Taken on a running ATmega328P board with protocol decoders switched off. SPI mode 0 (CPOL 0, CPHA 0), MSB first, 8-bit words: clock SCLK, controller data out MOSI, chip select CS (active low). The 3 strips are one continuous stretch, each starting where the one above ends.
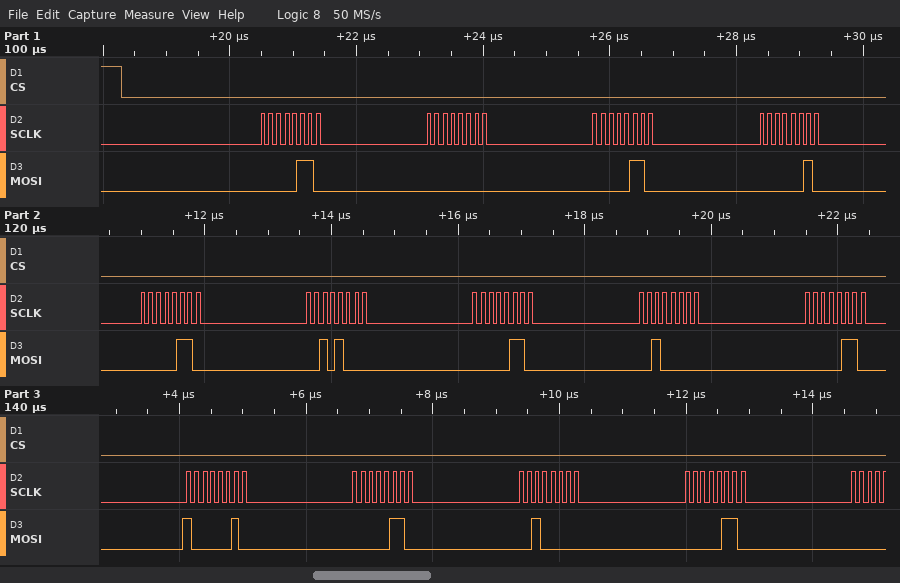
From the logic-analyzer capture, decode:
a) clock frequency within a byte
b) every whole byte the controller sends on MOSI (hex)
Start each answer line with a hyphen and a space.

- 8 MHz
- 06 00 06 02 06 28 06 20 06 82 06 20 06
